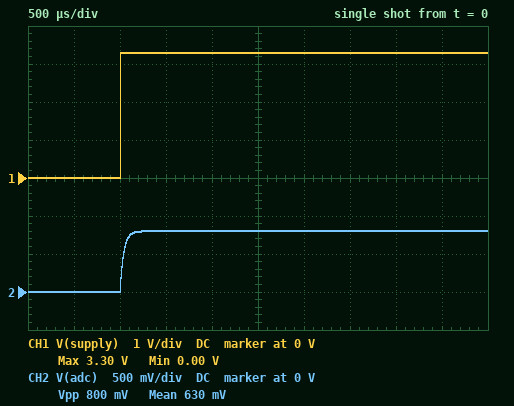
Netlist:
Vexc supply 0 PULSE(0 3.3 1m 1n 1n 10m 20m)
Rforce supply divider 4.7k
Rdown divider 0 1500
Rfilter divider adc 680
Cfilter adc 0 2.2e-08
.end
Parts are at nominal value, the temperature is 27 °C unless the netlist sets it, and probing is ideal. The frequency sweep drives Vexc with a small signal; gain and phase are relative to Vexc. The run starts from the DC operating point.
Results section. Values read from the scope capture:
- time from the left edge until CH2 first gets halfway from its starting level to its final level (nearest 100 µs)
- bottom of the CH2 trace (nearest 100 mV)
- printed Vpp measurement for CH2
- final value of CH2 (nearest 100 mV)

1.0 ms
0 V
800 mV
800 mV
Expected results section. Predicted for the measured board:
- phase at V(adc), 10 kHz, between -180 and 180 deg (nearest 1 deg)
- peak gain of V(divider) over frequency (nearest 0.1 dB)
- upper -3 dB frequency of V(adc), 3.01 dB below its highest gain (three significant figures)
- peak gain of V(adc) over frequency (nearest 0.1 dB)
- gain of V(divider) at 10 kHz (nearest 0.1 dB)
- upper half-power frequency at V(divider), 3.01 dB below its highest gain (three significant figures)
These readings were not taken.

-68 deg
-12.3 dB
3.98 kHz
-12.3 dB
-18.2 dB
4.69 kHz
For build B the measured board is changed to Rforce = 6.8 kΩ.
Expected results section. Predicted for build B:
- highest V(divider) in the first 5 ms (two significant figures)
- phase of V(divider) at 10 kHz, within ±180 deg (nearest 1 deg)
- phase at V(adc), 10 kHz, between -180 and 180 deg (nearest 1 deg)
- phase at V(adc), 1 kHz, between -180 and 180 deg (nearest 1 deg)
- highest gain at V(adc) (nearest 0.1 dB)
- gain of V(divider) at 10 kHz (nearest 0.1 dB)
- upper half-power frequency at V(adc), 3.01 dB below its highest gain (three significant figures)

600 mV
-26 deg
-69 deg
-15 deg
-14.9 dB
-21.1 dB
3.79 kHz
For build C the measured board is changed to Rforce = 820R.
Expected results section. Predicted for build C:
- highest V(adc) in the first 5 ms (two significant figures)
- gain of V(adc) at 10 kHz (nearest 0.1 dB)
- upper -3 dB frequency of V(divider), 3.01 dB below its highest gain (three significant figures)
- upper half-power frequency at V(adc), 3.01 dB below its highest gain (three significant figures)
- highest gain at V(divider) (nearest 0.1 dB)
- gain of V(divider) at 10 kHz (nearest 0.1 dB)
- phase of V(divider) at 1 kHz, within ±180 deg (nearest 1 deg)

2.1 V
-9.6 dB
9.85 kHz
5.98 kHz
-3.8 dB
-6.8 dB
-4 deg
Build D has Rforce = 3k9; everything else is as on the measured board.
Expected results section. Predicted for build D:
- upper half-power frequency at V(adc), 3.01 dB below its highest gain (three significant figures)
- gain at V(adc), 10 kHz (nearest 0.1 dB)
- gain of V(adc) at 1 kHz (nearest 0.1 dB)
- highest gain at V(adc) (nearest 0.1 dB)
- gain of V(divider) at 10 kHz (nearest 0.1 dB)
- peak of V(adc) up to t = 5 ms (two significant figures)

4.10 kHz
-19.5 dB
-11.4 dB
-11.1 dB
-16.8 dB
920 mV
